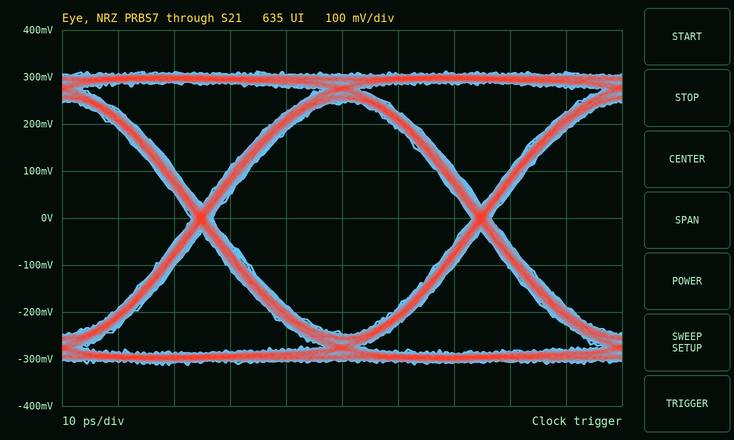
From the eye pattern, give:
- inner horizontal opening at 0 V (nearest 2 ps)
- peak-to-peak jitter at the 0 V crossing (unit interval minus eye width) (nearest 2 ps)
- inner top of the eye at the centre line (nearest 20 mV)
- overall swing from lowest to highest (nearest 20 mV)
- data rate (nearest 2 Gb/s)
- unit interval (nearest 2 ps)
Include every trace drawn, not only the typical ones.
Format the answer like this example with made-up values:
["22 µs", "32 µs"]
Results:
["46 ps", "4 ps", "240 mV", "620 mV", "20 Gb/s", "50 ps"]
